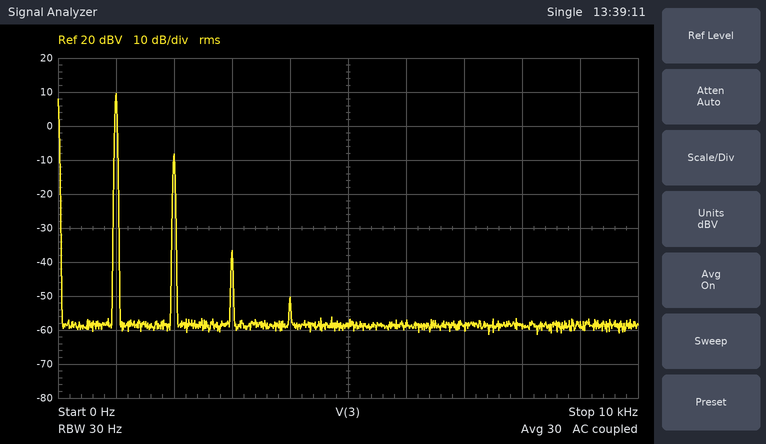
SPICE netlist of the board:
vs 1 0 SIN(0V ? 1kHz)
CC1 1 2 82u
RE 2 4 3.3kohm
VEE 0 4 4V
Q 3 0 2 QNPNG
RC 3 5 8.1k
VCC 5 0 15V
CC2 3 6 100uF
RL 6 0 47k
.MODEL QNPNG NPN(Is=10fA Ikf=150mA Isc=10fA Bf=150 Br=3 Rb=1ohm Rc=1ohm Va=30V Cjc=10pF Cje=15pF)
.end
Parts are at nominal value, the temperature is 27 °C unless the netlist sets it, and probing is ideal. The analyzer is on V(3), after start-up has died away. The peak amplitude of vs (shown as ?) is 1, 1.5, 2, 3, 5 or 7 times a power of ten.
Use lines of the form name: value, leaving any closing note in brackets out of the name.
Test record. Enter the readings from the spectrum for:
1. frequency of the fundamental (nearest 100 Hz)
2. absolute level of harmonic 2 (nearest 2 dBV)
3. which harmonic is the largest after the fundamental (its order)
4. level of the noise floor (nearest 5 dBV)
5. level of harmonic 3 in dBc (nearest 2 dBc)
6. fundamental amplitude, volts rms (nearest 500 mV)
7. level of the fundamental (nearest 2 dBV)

frequency of the fundamental: 1.0 kHz
absolute level of harmonic 2: -8 dBV
which harmonic is the largest after the fundamental: 2
level of the noise floor: -60 dBV
level of harmonic 3 in dBc: -46 dBc
fundamental amplitude, volts rms: 3.0 V
level of the fundamental: 10 dBV
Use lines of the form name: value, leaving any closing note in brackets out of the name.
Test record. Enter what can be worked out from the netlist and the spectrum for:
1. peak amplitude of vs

peak amplitude of vs: 20 mV
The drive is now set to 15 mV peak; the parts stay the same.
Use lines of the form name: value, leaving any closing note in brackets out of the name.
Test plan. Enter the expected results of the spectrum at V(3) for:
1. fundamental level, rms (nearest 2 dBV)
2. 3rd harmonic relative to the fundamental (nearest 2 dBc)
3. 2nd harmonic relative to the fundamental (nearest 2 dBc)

fundamental level, rms: 8 dBV
3rd harmonic relative to the fundamental: -52 dBc
2nd harmonic relative to the fundamental: -20 dBc
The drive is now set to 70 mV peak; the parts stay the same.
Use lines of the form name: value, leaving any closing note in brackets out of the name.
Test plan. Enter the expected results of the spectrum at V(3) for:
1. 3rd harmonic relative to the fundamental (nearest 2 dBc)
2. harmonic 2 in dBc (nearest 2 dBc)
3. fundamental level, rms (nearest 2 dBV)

3rd harmonic relative to the fundamental: -20 dBc
harmonic 2 in dBc: -12 dBc
fundamental level, rms: 16 dBV
